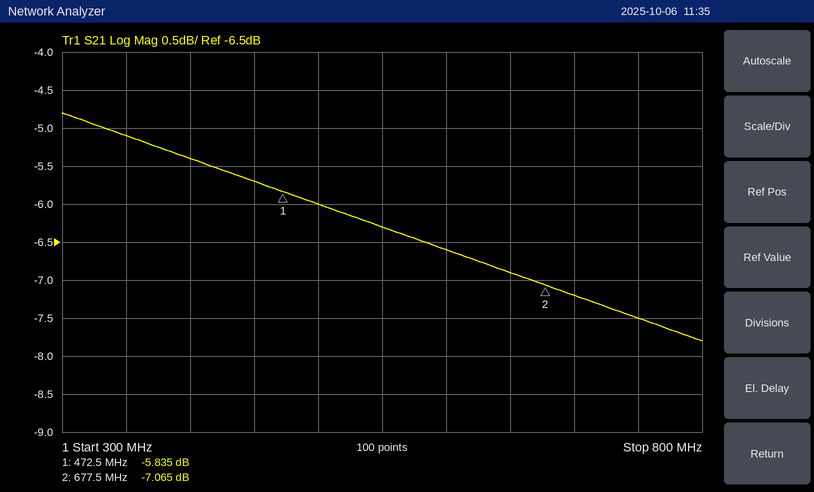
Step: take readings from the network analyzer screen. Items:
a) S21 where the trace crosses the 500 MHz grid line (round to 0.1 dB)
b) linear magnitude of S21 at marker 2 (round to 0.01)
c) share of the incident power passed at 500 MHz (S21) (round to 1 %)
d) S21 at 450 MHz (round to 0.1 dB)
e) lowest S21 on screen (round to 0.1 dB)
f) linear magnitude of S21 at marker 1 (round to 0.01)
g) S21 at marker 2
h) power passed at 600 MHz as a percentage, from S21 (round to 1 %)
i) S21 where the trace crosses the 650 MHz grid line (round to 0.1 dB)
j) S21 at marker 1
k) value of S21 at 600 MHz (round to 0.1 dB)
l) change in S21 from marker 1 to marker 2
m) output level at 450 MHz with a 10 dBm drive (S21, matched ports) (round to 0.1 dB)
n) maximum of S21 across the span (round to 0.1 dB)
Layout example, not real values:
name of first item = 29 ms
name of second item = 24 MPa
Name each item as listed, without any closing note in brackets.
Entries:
S21 where the trace crosses the 500 MHz grid line = -6.0 dB
linear magnitude of S21 at marker 2 = 0.44
share of the incident power passed at 500 MHz (S21) = 25 %
S21 at 450 MHz = -5.7 dB
lowest S21 on screen = -7.8 dB
linear magnitude of S21 at marker 1 = 0.51
S21 at marker 2 = -7.065 dB
power passed at 600 MHz as a percentage, from S21 = 22 %
S21 where the trace crosses the 650 MHz grid line = -6.9 dB
S21 at marker 1 = -5.835 dB
value of S21 at 600 MHz = -6.6 dB
change in S21 from marker 1 to marker 2 = -1.230 dB
output level at 450 MHz with a 10 dBm drive (S21, matched ports) = 4.3 dBm
maximum of S21 across the span = -4.8 dB
